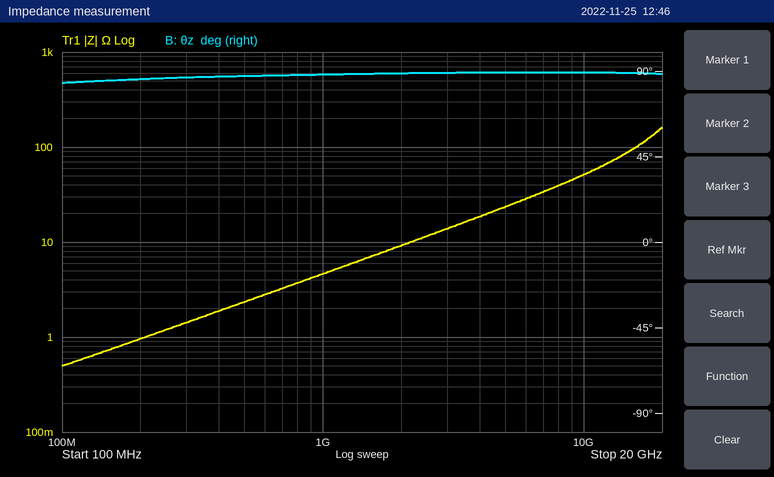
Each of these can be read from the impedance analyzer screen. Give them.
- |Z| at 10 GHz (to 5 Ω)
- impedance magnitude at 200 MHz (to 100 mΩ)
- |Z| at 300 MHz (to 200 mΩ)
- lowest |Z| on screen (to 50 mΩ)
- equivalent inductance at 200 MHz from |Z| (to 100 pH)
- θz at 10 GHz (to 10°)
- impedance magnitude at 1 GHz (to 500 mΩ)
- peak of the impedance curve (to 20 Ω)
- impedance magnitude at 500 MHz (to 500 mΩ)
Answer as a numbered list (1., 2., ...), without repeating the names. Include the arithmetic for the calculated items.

1. 50 Ω
2. 1.0 Ω
3. 1.4 Ω
4. 500 mΩ
5. L = 1.0 Ω/(2π × 200 MHz) ≈ 796 pH, so 800 pH to the nearest 100 pH
6. 90°
7. 4.5 Ω
8. 160 Ω
9. 2.5 Ω
